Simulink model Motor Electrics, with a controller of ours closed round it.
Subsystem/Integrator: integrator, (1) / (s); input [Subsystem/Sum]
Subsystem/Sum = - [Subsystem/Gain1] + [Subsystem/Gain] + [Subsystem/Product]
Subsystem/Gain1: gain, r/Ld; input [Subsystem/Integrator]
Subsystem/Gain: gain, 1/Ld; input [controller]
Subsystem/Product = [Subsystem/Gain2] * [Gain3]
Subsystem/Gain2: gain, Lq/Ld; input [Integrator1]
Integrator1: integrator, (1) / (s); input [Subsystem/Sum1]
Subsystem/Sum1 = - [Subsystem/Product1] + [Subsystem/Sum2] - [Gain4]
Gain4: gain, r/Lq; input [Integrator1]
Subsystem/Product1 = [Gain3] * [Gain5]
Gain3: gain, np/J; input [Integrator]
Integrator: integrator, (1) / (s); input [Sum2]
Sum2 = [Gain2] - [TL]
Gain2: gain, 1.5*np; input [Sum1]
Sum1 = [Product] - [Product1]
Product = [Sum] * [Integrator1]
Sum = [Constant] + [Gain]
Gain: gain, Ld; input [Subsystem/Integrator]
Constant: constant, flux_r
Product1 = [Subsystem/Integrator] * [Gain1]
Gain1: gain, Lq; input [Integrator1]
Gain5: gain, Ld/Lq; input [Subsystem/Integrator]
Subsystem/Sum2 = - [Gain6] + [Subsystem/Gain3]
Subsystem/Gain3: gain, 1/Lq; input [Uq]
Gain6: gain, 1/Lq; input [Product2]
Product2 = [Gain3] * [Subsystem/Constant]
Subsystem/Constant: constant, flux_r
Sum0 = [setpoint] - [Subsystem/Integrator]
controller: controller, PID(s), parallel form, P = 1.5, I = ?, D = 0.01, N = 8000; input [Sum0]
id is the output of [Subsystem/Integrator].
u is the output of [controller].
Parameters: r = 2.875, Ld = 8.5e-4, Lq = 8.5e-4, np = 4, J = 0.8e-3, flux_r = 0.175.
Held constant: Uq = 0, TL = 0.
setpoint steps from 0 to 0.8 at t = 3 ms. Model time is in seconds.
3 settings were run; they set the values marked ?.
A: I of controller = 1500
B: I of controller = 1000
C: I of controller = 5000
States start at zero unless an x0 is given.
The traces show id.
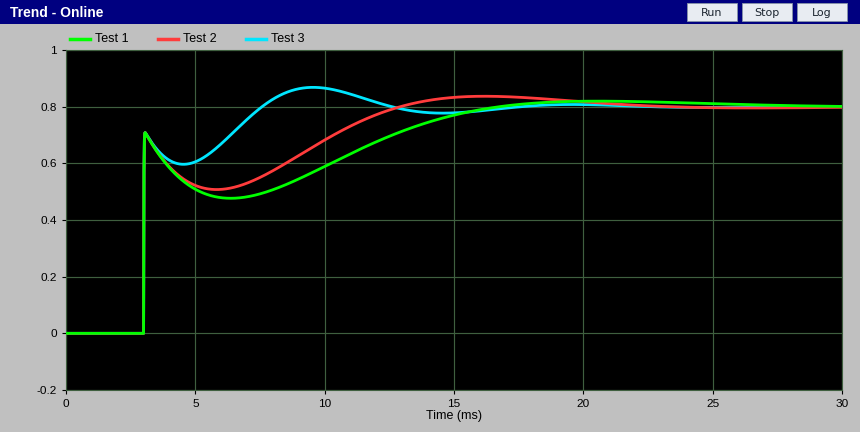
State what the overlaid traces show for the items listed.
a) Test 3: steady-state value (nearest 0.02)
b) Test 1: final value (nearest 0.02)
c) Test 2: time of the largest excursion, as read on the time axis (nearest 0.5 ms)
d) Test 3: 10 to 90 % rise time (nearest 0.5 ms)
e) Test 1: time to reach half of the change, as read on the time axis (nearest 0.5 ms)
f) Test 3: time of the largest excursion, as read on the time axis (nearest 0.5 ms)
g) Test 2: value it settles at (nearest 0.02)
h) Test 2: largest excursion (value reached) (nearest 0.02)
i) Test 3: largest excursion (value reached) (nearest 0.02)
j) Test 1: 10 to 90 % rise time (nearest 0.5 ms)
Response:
0.80
0.80
16.0 ms
3.5 ms
3.0 ms
9.5 ms
0.80
0.84
0.86
10.0 ms
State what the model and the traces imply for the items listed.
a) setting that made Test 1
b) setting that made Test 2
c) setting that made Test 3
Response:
B
A
C
